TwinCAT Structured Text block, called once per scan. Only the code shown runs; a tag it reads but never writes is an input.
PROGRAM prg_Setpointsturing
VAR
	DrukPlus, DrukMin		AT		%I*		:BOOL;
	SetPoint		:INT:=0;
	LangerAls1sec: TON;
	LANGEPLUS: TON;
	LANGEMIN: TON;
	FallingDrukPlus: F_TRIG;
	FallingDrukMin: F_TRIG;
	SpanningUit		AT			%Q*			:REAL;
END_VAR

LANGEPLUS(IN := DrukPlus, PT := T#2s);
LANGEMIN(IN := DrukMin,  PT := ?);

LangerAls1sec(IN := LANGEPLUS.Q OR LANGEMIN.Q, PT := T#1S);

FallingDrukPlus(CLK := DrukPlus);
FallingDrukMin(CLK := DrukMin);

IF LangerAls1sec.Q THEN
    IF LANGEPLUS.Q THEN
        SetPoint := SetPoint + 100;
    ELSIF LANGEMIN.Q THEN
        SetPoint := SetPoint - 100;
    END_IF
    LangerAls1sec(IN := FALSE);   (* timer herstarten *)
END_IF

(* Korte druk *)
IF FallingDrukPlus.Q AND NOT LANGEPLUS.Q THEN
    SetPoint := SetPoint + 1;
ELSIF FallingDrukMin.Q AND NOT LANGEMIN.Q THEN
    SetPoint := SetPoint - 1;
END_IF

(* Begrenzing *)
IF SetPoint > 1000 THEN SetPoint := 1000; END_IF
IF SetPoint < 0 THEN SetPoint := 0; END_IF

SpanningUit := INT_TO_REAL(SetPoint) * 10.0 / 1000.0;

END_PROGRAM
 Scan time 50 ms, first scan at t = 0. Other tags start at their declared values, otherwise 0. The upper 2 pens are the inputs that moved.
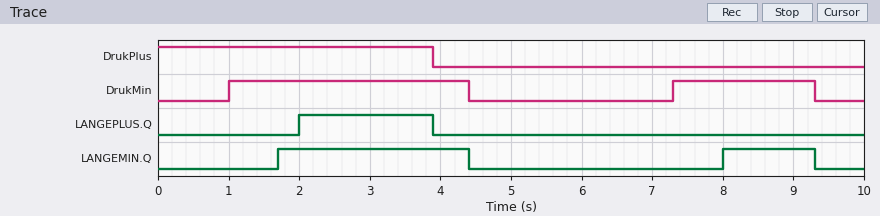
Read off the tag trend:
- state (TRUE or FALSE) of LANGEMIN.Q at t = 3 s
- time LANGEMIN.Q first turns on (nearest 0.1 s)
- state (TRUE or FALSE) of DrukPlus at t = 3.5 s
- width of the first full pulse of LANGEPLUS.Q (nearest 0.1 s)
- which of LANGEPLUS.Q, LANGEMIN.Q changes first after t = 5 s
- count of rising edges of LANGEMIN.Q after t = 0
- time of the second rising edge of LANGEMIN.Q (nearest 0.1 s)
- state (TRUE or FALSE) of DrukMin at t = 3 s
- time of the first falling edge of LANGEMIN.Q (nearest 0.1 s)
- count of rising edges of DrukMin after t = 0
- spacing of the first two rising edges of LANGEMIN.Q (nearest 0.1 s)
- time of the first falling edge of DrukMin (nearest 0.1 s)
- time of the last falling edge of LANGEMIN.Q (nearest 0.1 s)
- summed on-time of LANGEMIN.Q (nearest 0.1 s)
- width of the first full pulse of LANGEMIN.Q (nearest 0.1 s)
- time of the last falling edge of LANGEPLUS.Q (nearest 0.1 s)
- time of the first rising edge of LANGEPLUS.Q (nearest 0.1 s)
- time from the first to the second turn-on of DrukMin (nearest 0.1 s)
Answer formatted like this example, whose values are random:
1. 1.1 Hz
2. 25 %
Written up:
1. TRUE
2. 1.7 s
3. TRUE
4. 1.9 s
5. LANGEMIN.Q
6. 2
7. 8.0 s
8. TRUE
9. 4.4 s
10. 2
11. 6.3 s
12. 4.4 s
13. 9.3 s
14. 4.0 s
15. 2.7 s
16. 3.9 s
17. 2.0 s
18. 6.3 s
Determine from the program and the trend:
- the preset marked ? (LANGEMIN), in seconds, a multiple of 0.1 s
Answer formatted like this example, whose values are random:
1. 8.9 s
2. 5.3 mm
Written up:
1. 0.7 s
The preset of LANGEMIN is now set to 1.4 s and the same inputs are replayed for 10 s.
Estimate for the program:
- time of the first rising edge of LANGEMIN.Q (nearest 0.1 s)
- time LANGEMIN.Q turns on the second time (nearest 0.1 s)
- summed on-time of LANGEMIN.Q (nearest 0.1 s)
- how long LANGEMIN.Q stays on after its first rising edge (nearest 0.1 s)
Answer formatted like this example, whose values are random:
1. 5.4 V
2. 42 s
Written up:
1. 2.4 s
2. 8.7 s
3. 2.6 s
4. 2.0 s
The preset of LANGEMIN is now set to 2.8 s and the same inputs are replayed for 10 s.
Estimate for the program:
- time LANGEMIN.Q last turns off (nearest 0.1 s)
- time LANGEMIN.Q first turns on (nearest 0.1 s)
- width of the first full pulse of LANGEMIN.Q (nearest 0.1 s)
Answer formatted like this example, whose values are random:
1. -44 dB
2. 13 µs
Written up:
1. 4.4 s
2. 3.8 s
3. 0.6 s
